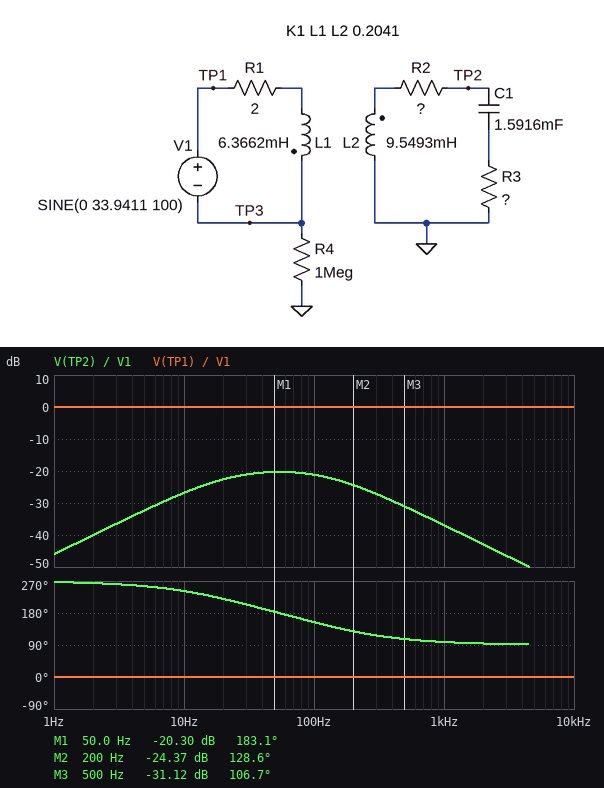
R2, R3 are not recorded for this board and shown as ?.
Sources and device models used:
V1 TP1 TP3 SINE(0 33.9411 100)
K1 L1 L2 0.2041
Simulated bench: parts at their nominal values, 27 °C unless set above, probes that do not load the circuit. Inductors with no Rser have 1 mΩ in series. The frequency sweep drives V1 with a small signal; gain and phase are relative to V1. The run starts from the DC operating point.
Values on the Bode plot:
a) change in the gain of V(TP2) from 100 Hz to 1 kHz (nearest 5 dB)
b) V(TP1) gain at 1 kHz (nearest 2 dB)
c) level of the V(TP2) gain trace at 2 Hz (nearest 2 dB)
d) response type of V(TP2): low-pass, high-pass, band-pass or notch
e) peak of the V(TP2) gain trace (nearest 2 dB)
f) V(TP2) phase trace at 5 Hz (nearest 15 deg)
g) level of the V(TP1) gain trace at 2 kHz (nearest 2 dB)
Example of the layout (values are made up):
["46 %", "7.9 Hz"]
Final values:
["-15 dB", "0 dB", "-40 dB", "band-pass", "-20 dB", "255 deg", "0 dB"]
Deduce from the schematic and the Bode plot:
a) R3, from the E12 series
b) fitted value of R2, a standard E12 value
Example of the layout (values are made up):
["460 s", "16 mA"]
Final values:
["3.3 Ω", "2.2 Ω"]
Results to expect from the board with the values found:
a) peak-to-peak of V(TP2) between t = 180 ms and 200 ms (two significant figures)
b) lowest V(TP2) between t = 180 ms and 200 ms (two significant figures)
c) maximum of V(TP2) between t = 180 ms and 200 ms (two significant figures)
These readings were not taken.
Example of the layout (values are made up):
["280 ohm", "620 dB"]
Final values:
["5.9 V", "-3.0 V", "3.0 V"]
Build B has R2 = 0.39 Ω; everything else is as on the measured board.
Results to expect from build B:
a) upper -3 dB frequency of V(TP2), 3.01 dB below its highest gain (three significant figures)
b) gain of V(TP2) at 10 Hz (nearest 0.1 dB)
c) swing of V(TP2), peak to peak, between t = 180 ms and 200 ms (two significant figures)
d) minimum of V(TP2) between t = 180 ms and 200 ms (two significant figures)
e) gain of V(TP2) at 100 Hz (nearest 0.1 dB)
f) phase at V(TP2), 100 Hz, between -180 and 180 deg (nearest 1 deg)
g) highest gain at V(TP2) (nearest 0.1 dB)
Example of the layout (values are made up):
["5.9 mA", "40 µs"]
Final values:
["122 Hz", "-26.2 dB", "7.9 V", "-3.9 V", "-18.7 dB", "144 deg", "-16.9 dB"]
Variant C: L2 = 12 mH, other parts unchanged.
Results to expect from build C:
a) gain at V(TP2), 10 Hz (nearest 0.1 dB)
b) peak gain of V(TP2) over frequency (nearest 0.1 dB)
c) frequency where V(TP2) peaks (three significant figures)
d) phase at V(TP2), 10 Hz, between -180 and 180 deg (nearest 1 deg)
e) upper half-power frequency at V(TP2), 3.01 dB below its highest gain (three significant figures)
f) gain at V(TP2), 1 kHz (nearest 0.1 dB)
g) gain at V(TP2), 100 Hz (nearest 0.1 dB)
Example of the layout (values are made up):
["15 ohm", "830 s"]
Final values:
["-23.8 dB", "-17.7 dB", "38.3 Hz", "-119 deg", "95.2 Hz", "-39.6 dB", "-21.0 dB"]
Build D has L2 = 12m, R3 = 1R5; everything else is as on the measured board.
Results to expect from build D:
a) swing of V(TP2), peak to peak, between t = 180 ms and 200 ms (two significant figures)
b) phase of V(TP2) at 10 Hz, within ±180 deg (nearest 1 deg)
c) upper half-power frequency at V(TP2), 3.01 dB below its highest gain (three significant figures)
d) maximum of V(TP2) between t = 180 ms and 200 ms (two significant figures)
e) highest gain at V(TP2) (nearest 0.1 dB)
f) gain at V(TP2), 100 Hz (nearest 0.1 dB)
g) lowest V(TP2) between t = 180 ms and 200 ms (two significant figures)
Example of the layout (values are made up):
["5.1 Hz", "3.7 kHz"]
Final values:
["3.6 V", "-120 deg", "57.1 Hz", "1.8 V", "-16.9 dB", "-25.4 dB", "-1.8 V"]
